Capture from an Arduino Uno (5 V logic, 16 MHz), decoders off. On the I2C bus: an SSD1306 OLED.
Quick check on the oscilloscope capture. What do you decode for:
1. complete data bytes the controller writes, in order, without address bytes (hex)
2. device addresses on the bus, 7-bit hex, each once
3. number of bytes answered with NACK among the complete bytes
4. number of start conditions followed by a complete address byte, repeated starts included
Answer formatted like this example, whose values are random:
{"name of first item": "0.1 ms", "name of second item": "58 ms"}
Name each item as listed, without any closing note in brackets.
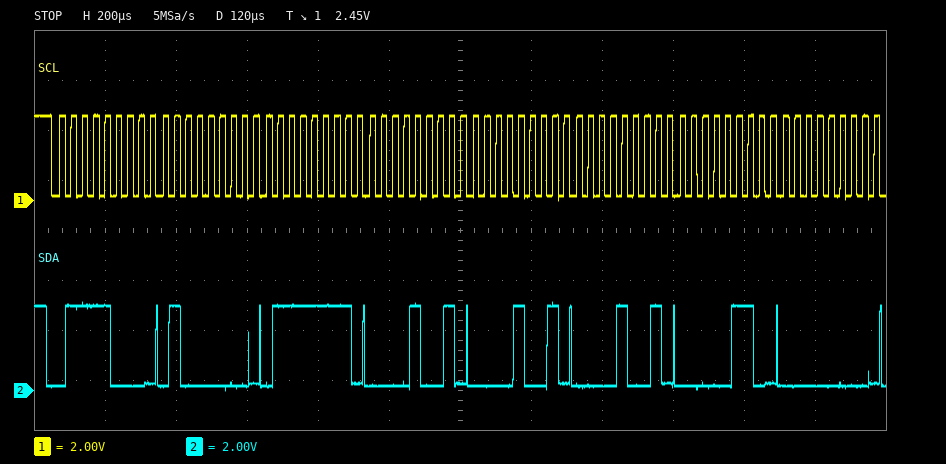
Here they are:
{"complete data bytes the controller writes, in order, without address bytes": "40 7F 09 09 09 06 00", "device addresses on the bus, 7-bit hex, each once": "0x3C", "number of bytes answered with NACK among the complete bytes": "0", "number of start conditions followed by a complete address byte, repeated starts included": "1"}
